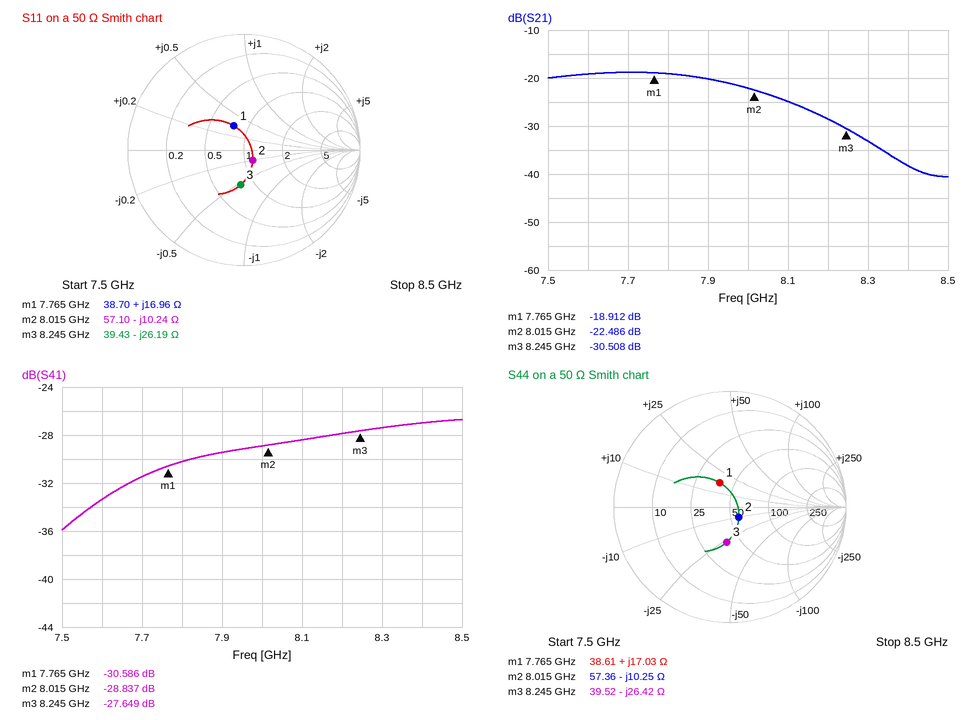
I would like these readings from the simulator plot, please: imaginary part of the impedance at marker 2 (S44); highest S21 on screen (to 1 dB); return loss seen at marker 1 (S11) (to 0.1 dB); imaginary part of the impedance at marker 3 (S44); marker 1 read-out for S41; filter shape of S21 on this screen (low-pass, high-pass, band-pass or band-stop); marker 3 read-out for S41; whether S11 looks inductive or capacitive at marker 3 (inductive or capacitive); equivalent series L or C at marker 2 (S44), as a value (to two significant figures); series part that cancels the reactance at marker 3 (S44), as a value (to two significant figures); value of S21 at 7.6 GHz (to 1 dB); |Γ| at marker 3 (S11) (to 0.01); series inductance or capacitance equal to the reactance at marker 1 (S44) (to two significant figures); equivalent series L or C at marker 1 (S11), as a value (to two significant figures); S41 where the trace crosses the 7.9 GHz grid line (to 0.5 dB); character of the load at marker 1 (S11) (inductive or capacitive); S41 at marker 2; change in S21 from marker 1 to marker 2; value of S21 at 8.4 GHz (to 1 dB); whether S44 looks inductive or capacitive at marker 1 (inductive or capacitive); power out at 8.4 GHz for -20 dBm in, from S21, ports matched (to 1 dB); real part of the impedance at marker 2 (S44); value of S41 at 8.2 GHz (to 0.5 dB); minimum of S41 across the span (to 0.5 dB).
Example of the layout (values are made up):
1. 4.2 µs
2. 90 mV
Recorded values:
1. -10.25 Ω
2. -19 dB
3. 12.9 dB
4. -26.42 Ω
5. -30.586 dB
6. low-pass
7. -27.649 dB
8. capacitive
9. 1.9 pF
10. 510 pH
11. -19 dB
12. 0.30
13. 350 pH
14. 350 pH
15. -29.5 dB
16. inductive
17. -28.837 dB
18. -3.574 dB
19. -38 dB
20. inductive
21. -58 dBm
22. 57.36 Ω
23. -28.0 dB
24. -36.0 dB
